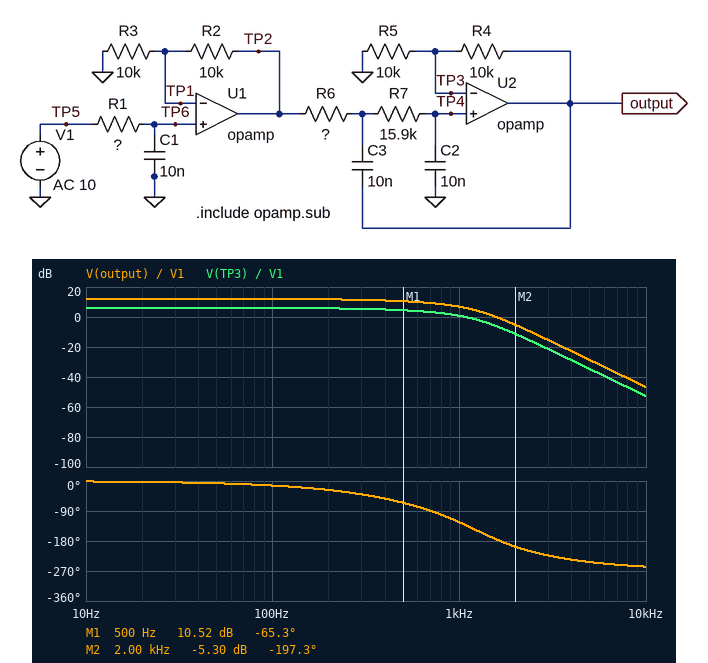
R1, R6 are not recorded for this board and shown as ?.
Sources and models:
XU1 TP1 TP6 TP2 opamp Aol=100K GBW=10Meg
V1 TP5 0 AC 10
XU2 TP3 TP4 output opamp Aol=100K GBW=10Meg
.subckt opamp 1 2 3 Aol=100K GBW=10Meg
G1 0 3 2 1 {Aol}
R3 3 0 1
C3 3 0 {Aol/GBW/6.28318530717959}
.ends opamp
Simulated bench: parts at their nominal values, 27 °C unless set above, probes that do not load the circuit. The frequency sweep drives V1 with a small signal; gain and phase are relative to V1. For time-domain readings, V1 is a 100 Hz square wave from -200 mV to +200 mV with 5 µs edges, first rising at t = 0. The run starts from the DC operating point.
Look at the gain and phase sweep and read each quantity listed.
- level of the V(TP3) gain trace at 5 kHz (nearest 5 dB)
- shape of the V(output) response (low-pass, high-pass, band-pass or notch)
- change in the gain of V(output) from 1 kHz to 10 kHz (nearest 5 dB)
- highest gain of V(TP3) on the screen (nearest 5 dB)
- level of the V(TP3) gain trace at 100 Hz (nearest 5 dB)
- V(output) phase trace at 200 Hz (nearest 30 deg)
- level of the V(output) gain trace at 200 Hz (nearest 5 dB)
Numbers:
-35 dB
low-pass
-55 dB
5 dB
5 dB
-30 deg
10 dB
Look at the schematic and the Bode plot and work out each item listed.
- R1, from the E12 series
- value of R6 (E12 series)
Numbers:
22 kΩ
10 kΩ
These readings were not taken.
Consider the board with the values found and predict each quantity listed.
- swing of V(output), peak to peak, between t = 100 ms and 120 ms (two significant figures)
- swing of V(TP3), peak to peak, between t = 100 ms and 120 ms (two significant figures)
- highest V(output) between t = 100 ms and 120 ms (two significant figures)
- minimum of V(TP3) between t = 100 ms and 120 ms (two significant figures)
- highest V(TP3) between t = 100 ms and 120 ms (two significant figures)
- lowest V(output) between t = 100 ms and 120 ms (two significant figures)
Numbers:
1.6 V
800 mV
800 mV
-400 mV
400 mV
-800 mV
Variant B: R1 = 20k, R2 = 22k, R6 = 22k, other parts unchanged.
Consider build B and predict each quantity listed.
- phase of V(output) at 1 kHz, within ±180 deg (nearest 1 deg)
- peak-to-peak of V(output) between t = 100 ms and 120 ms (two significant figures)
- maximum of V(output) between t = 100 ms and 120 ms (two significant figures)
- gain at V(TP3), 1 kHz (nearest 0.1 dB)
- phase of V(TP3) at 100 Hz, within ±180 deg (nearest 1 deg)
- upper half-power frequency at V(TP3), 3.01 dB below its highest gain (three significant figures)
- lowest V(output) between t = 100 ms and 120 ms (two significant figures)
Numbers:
-162 deg
3.1 V
1.6 V
5.4 dB
-13 deg
902 Hz
-1.6 V
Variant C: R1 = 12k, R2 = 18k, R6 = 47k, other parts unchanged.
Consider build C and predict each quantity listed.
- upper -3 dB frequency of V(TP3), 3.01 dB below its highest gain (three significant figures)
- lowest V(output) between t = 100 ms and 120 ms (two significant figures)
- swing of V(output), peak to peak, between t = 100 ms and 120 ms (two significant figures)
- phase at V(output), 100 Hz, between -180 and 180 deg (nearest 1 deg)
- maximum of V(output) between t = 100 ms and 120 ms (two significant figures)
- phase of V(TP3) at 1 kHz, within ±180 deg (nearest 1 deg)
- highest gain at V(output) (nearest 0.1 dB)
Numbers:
674 Hz
-1.9 V
3.8 V
-10 deg
1.9 V
170 deg
19.4 dB
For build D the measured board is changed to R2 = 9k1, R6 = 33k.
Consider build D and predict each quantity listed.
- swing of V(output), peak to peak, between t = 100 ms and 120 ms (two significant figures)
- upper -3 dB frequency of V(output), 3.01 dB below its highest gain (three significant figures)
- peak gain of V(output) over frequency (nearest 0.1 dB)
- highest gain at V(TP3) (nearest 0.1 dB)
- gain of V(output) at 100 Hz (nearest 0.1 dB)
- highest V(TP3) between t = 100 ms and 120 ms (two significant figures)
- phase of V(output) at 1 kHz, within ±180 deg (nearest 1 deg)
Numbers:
2.1 V
772 Hz
13.2 dB
7.2 dB
11.7 dB
530 mV
169 deg
